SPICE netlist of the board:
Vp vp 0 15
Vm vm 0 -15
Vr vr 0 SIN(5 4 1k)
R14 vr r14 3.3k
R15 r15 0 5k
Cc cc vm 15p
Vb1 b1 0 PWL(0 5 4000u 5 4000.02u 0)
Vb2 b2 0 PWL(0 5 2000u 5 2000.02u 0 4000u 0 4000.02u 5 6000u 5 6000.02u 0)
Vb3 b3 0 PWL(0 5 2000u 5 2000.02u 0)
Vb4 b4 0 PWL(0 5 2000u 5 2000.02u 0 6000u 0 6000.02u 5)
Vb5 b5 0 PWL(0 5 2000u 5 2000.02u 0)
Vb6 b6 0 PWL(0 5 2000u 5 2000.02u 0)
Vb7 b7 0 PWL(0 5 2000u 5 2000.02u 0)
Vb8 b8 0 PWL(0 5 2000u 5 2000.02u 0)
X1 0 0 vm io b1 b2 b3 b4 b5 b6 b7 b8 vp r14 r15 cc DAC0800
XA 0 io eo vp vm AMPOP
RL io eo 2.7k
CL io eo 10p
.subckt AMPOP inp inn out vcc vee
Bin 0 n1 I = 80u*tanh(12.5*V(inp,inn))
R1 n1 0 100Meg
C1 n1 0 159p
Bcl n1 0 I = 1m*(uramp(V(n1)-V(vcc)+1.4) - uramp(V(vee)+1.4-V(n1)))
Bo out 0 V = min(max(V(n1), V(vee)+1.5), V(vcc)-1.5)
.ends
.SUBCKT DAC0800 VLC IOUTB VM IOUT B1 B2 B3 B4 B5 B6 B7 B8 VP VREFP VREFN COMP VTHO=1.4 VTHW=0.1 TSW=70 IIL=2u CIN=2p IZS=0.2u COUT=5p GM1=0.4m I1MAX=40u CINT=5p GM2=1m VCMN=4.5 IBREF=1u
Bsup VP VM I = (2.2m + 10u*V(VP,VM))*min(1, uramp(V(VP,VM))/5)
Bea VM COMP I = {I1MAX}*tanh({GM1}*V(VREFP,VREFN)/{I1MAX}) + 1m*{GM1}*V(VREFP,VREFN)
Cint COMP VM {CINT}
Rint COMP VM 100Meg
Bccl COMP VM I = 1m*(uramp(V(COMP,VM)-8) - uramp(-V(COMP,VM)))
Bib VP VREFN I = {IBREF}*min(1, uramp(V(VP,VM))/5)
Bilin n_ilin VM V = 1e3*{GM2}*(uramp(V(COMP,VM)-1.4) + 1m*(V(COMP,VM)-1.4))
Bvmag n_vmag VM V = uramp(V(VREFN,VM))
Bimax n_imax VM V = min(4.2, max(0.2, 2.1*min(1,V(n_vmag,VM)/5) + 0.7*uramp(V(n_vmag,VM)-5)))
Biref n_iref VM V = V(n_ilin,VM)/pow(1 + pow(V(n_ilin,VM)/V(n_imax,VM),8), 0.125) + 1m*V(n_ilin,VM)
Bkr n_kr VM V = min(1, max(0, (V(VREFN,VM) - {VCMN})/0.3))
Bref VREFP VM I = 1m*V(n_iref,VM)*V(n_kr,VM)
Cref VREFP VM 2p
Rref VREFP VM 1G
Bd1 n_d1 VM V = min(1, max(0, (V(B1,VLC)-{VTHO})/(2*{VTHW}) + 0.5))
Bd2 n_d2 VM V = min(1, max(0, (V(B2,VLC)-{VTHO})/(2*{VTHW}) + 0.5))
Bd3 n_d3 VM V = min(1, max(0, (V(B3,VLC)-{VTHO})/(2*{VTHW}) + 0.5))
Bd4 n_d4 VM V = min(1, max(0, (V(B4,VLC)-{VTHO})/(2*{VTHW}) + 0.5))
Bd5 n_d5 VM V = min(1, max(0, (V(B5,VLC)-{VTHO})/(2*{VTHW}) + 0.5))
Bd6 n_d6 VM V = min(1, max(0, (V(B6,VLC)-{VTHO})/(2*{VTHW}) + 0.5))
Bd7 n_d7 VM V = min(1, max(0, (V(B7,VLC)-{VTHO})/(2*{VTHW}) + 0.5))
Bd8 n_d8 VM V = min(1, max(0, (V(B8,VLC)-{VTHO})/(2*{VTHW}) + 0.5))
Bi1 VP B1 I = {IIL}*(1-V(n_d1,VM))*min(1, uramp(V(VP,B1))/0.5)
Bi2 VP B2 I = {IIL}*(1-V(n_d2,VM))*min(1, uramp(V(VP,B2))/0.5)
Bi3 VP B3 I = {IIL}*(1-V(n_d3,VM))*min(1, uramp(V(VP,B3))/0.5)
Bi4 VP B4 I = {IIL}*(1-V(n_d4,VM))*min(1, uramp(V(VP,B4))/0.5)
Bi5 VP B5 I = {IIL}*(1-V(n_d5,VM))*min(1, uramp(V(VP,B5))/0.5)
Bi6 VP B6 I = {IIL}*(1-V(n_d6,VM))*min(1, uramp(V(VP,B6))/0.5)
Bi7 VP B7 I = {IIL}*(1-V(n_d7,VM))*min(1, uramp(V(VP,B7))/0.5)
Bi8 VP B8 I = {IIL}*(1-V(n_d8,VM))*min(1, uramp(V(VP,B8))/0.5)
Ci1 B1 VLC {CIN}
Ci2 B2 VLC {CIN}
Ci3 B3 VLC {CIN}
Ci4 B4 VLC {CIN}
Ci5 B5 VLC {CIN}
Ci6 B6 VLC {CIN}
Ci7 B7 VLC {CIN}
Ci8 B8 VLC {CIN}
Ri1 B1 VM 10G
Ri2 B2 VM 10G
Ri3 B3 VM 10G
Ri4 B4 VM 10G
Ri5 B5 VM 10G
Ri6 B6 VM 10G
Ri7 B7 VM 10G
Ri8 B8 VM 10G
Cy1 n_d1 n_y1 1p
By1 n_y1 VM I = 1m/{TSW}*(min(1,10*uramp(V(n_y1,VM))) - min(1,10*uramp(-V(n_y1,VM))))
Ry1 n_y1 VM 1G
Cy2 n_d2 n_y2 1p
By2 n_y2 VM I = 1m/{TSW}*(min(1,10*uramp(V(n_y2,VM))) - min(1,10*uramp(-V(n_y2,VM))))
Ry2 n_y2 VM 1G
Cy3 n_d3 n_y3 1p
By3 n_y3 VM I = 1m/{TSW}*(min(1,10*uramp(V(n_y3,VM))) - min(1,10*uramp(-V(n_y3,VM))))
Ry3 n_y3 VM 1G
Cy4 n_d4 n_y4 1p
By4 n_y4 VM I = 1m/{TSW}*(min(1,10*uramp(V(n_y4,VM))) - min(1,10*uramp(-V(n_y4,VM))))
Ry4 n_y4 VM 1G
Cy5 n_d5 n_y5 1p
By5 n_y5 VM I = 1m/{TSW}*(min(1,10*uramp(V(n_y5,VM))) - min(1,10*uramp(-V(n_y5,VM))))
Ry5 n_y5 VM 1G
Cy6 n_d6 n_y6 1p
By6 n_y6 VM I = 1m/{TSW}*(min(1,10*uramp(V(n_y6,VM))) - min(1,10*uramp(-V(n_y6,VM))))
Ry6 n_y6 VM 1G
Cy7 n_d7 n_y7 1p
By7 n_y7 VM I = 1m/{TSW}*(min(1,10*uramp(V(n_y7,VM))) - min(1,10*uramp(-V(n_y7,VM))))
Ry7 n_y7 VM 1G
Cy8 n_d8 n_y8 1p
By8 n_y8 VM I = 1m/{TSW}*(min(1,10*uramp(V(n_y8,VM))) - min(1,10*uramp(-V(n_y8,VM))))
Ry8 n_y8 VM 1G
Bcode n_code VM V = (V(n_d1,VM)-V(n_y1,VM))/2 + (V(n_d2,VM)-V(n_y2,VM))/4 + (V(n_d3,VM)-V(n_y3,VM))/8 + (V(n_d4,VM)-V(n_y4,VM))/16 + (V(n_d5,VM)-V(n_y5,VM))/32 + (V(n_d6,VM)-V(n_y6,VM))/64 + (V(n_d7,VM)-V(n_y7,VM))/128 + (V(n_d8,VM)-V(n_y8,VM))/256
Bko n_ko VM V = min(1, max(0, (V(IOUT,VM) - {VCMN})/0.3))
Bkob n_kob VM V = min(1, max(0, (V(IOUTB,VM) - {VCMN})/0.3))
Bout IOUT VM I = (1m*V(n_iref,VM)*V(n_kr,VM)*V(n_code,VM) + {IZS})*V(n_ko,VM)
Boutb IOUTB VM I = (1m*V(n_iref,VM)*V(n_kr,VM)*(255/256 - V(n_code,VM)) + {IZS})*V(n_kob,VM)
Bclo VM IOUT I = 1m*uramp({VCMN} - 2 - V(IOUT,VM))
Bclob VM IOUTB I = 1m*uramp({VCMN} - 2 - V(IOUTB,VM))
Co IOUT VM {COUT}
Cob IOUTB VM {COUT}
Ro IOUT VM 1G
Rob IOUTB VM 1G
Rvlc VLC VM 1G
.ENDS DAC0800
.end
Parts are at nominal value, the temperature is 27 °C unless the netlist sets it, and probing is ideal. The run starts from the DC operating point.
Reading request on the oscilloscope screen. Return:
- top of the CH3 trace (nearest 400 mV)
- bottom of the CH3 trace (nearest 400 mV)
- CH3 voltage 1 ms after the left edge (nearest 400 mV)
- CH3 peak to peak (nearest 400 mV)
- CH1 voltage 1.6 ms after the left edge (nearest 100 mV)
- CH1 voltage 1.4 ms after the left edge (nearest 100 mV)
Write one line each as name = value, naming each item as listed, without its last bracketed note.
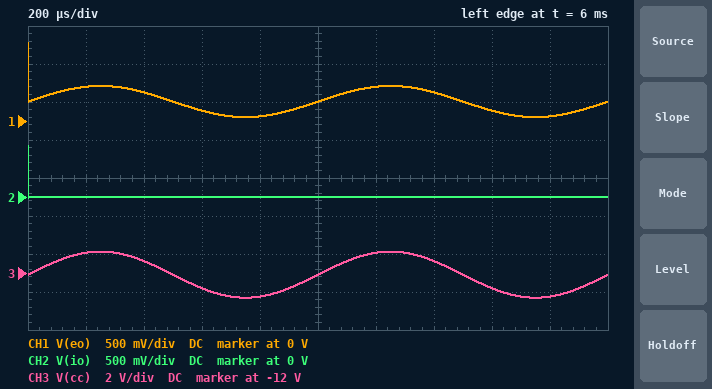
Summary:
top of the CH3 trace = -10.8 V
bottom of the CH3 trace = -13.2 V
CH3 voltage 1 ms after the left edge = -12.0 V
CH3 peak to peak = 2.4 V
CH1 voltage 1.6 ms after the left edge = 100 mV
CH1 voltage 1.4 ms after the left edge = 400 mV
